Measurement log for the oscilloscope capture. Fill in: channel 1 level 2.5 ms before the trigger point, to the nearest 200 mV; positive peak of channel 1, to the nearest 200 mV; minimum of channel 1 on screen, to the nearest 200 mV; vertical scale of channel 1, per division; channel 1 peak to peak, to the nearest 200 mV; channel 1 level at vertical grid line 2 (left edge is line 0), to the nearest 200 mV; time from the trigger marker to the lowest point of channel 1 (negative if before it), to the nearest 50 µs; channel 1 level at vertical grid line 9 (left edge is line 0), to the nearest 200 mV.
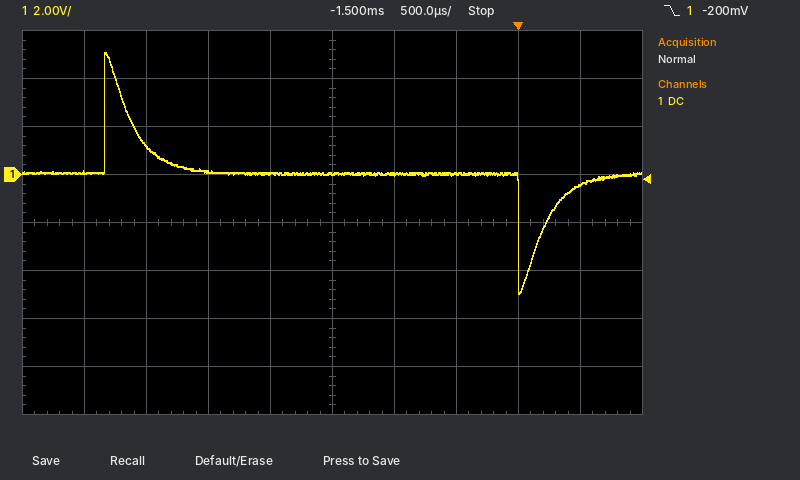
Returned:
200 mV
5.0 V
-5.0 V
2 V
10.0 V
1.2 V
0 µs
-400 mV
